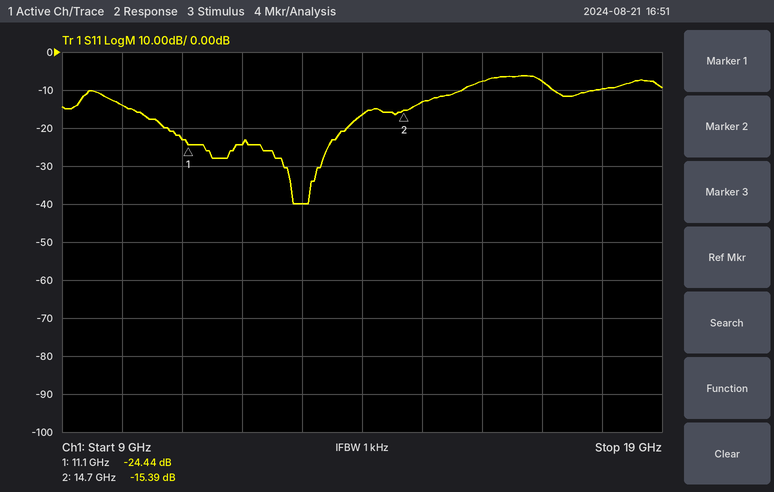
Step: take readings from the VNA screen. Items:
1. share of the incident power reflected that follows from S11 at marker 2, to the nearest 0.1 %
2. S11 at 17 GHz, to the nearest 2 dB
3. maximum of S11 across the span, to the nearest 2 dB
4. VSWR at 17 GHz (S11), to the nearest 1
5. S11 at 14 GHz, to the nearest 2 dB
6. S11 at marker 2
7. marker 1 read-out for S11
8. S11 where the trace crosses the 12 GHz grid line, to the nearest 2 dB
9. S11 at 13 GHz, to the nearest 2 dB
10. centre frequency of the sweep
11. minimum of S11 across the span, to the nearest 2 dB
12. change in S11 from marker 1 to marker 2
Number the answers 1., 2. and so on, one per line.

1. 2.9 %
2. -8 dB
3. -6 dB
4. 2
5. -16 dB
6. -15.39 dB
7. -24.44 dB
8. -24 dB
9. -40 dB
10. 14 GHz
11. -40 dB
12. 9.05 dB
